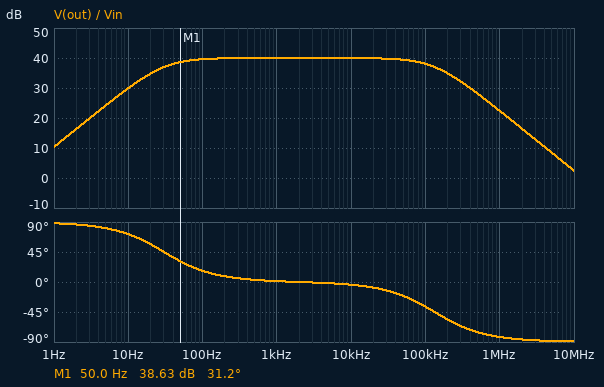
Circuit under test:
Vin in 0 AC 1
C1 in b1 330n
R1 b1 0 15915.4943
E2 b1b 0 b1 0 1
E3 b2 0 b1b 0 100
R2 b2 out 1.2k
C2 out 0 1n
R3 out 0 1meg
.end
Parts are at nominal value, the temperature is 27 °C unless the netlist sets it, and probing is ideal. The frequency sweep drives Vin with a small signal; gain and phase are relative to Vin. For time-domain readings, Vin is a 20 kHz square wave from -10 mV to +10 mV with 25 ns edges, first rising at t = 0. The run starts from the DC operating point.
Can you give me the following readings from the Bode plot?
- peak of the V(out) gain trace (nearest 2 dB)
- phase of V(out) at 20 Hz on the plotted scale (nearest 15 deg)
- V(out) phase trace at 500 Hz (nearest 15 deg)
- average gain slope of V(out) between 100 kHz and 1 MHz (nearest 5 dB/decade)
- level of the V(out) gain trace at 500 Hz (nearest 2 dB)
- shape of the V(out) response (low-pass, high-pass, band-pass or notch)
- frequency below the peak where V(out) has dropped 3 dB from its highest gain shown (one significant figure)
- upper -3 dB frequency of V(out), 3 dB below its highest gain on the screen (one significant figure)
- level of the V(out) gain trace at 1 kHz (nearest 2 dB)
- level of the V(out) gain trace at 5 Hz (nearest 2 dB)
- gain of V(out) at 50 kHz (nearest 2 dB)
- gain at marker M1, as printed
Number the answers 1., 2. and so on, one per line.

1. 40 dB
2. 60 deg
3. 0 deg
4. -15 dB/decade
5. 40 dB
6. band-pass
7. 30 Hz
8. 100 kHz
9. 40 dB
10. 24 dB
11. 40 dB
12. 38.63 dB
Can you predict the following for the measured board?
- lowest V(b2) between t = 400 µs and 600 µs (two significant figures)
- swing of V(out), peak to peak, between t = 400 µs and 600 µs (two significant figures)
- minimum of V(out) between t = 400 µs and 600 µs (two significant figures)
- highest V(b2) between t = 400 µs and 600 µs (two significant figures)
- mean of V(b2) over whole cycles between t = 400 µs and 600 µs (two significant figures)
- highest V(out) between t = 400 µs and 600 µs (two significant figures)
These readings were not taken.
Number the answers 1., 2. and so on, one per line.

1. -110 mV
2. 2.0 V
3. -110 mV
4. 1.9 V
5. 910 mV
6. 1.9 V
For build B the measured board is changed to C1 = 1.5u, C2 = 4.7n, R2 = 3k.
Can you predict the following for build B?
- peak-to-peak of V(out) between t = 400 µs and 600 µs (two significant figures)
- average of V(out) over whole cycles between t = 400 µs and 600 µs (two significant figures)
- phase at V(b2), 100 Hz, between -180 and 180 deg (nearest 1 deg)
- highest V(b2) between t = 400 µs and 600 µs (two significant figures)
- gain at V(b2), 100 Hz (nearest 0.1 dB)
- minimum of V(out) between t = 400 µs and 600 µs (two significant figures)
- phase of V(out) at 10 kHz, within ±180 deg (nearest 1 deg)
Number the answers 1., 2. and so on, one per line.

1. 1.4 V
2. 980 mV
3. 4 deg
4. 2.0 V
5. 40.0 dB
6. 260 mV
7. -41 deg
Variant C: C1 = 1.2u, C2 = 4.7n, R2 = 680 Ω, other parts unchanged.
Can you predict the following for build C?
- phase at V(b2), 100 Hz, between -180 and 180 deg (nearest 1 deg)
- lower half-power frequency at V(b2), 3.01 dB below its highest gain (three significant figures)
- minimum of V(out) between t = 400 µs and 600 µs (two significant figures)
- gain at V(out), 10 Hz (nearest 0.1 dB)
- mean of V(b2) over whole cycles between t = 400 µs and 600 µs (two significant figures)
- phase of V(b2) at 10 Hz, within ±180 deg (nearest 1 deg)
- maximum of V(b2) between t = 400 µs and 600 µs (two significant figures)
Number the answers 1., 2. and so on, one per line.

1. 5 deg
2. 8.33 Hz
3. -30 mV
4. 37.7 dB
5. 970 mV
6. 40 deg
7. 2.0 V
